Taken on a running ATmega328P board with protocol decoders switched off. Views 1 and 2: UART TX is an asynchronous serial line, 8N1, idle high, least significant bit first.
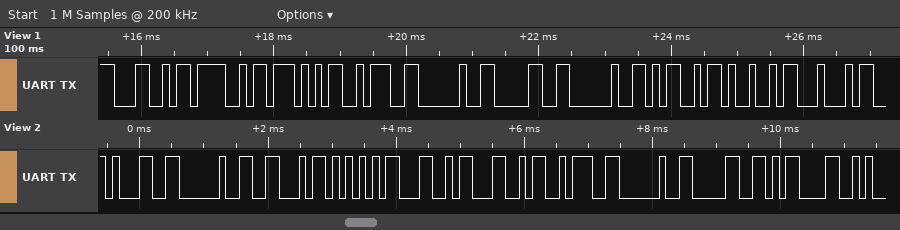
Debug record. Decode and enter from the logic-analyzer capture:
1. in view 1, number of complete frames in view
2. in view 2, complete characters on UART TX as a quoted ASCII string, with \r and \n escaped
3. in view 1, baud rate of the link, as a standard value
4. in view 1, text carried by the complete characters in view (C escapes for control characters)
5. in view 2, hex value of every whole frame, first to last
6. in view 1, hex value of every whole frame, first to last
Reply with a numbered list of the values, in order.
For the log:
1. 10
2. "1 FULL: 0\r"
3. 9600 baud
4. "LOW: 0 MID"
5. 0x31 0x20 0x46 0x55 0x4C 0x4C 0x3A 0x20 0x30 0x0D
6. 0x4C 0x4F 0x57 0x3A 0x20 0x30 0x20 0x4D 0x49 0x44
